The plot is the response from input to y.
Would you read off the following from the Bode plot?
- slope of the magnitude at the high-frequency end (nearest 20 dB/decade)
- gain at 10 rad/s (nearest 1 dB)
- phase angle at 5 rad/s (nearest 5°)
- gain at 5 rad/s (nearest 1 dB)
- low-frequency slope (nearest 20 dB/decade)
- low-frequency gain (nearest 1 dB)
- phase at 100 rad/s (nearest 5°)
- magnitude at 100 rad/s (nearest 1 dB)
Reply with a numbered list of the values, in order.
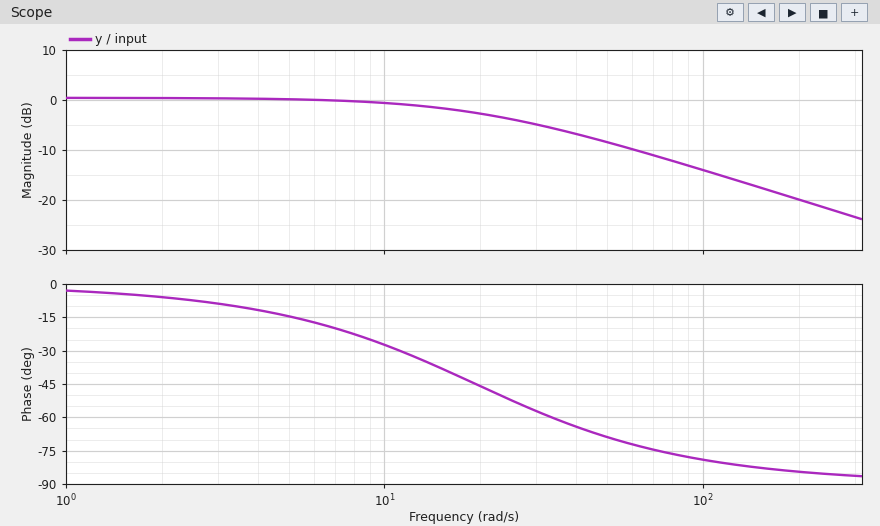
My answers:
1. -20 dB/decade
2. -1 dB
3. -15°
4. 0 dB
5. 0 dB/decade
6. 0 dB
7. -80°
8. -14 dB
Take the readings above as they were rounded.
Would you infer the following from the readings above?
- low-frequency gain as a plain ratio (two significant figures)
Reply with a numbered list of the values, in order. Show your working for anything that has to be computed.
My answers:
1. 10^(0 / 20) = 1.0
